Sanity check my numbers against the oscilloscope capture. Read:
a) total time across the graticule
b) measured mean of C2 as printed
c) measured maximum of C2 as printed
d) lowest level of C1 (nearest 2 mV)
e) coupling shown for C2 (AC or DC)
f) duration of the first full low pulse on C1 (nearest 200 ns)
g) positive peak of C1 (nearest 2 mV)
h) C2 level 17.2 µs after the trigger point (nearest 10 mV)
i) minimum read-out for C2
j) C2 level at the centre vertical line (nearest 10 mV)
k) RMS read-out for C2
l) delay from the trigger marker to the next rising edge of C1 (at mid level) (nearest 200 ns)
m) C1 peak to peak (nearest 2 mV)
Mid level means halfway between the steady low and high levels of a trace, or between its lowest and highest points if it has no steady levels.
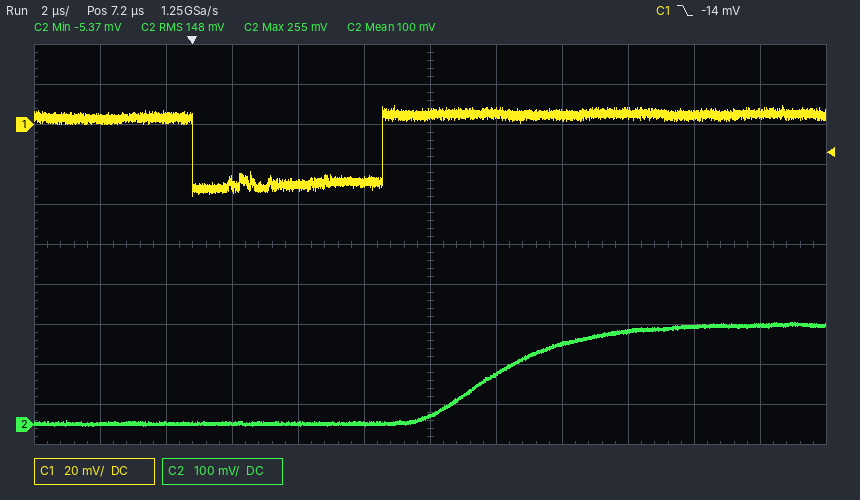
24 µs
100 mV
255 mV
-36 mV
DC
5.8 µs
10 mV
250 mV
-5.37 mV
20 mV
148 mV
5.8 µs
46 mV
